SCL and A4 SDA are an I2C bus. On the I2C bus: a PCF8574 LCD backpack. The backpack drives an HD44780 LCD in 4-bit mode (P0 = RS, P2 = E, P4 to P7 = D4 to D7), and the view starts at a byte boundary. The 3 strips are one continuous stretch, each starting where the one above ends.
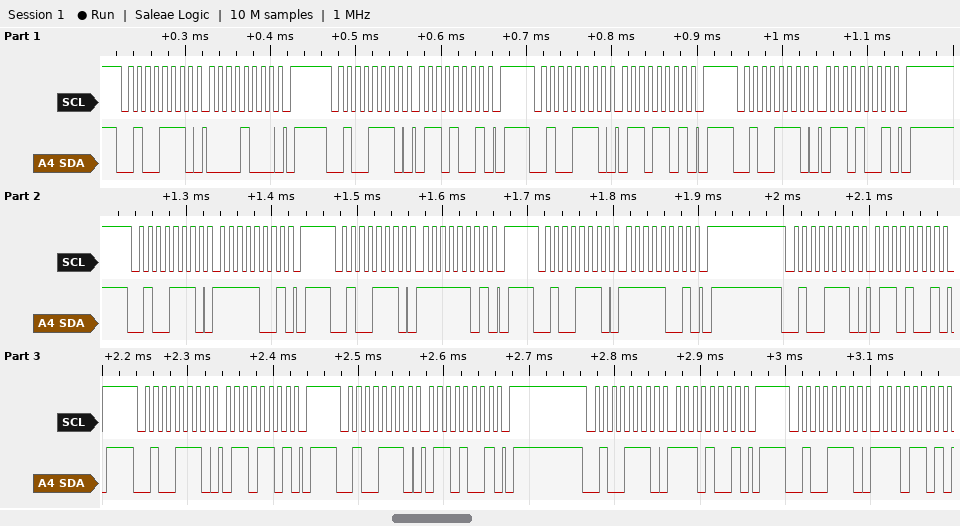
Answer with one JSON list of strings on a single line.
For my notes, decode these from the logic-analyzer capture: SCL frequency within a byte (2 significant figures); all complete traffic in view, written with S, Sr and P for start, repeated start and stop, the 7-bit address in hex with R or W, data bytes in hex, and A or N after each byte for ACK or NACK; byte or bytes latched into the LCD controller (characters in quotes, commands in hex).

["100 kHz", "S 27W A 08 A P S 27W A 69 A P S 27W A 6D A P S 27W A 69 A P S 27W A F9 A P S 27W A FD A P S 27W A F9 A P S 27W A 69 A P S 27W A 6D A P S 27W A 69 A P S 27W A E9 A P S 27W A ED A", "'o'"]
